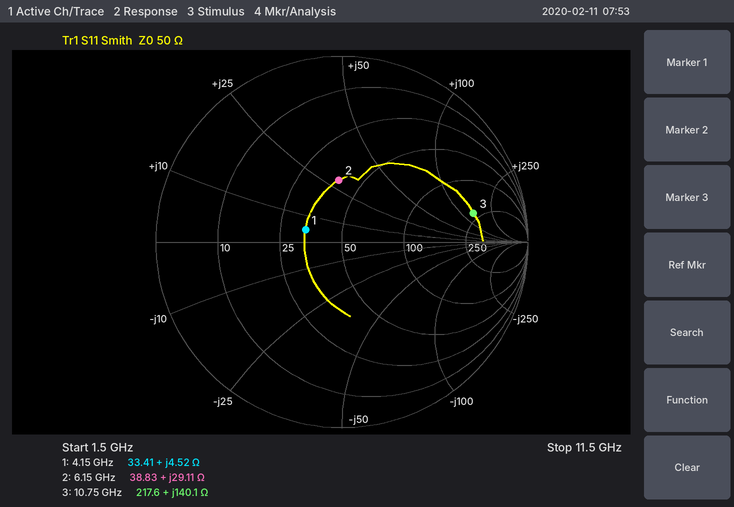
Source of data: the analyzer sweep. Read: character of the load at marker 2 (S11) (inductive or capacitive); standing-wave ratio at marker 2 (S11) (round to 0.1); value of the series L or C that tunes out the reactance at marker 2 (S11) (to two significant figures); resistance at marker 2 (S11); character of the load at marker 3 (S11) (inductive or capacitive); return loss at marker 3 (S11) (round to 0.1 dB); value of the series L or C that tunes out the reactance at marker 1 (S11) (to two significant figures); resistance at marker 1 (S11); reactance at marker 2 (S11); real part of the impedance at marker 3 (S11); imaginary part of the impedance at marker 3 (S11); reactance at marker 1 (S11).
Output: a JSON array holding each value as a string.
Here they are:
["inductive", "2.0", "890 fF", "38.83 Ω", "inductive", "2.8 dB", "8.5 pF", "33.41 Ω", "+29.11 Ω", "217.6 Ω", "+140.1 Ω", "+4.52 Ω"]
